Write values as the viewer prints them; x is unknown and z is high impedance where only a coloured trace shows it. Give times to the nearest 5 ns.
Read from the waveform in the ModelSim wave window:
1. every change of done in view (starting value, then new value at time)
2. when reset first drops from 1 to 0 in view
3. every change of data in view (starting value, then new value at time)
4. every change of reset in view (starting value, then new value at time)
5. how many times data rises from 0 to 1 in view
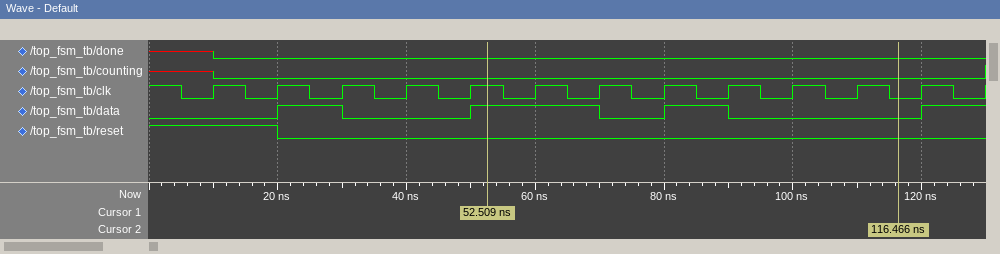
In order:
x, 0 at 10 ns
20 ns
0, 1 at 20 ns, 0 at 30 ns, 1 at 50 ns, 0 at 70 ns, 1 at 80 ns, 0 at 90 ns, 1 at 120 ns
1, 0 at 20 ns
4
